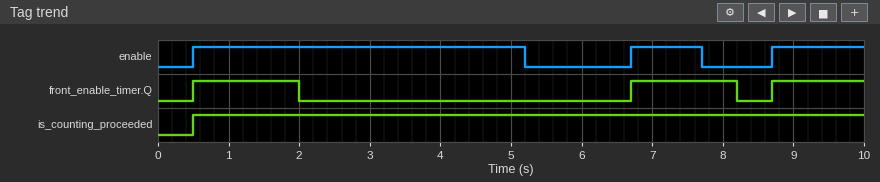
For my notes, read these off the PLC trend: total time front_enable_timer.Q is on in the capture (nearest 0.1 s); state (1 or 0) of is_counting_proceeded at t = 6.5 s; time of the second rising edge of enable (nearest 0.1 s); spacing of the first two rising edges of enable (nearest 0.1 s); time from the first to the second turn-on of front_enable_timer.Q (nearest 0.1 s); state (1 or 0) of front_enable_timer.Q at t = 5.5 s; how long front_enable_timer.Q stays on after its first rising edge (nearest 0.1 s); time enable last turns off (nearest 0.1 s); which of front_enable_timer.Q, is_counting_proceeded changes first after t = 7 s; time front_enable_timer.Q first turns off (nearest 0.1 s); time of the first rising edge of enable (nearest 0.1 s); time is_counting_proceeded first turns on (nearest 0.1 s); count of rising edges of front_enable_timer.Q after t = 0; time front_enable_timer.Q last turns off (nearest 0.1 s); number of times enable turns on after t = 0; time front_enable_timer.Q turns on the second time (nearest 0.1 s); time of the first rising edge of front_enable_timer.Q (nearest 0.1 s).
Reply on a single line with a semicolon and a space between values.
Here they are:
4.3 s; 1; 6.7 s; 6.2 s; 6.2 s; 0; 1.5 s; 7.7 s; front_enable_timer.Q; 2.0 s; 0.5 s; 0.5 s; 3; 8.2 s; 3; 6.7 s; 0.5 s
